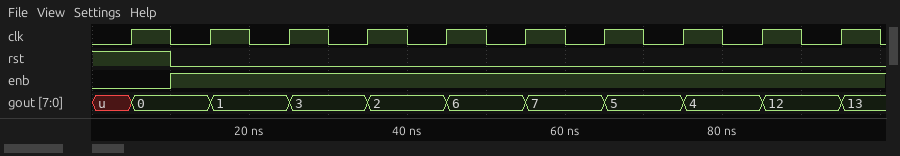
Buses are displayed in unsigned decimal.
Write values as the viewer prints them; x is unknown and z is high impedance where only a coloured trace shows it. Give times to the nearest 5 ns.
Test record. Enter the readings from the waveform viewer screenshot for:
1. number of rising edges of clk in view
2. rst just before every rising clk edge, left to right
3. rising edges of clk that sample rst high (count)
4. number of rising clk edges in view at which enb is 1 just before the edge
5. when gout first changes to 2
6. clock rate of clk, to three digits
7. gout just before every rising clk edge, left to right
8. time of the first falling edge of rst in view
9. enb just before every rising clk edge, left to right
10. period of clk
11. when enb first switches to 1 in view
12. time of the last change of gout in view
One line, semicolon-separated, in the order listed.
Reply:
10; 1 0 0 0 0 0 0 0 0 0; 1; 9; 35 ns; 100 MHz; u, 0, 1, 3, 2, 6, 7, 5, 4, 12; 10 ns; 0 1 1 1 1 1 1 1 1 1; 10 ns; 10 ns; 95 ns
